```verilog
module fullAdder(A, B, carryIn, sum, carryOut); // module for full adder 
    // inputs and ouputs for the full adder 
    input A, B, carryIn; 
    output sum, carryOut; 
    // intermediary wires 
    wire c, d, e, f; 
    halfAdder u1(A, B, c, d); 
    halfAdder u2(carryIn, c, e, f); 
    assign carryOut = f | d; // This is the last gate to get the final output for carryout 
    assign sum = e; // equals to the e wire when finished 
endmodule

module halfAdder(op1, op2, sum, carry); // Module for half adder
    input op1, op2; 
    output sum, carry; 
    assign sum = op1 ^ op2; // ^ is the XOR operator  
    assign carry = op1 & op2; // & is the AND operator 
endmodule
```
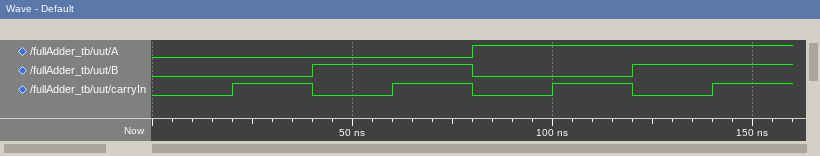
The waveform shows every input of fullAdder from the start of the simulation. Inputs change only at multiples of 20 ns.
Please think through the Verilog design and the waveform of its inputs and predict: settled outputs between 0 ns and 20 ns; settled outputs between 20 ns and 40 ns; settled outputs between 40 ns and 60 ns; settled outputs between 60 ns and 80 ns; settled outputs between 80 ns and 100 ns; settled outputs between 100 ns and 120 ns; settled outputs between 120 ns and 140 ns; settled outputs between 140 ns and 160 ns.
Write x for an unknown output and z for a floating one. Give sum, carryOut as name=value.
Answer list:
sum=0, carryOut=0
sum=1, carryOut=0
sum=1, carryOut=0
sum=0, carryOut=1
sum=1, carryOut=0
sum=0, carryOut=1
sum=0, carryOut=1
sum=1, carryOut=1
